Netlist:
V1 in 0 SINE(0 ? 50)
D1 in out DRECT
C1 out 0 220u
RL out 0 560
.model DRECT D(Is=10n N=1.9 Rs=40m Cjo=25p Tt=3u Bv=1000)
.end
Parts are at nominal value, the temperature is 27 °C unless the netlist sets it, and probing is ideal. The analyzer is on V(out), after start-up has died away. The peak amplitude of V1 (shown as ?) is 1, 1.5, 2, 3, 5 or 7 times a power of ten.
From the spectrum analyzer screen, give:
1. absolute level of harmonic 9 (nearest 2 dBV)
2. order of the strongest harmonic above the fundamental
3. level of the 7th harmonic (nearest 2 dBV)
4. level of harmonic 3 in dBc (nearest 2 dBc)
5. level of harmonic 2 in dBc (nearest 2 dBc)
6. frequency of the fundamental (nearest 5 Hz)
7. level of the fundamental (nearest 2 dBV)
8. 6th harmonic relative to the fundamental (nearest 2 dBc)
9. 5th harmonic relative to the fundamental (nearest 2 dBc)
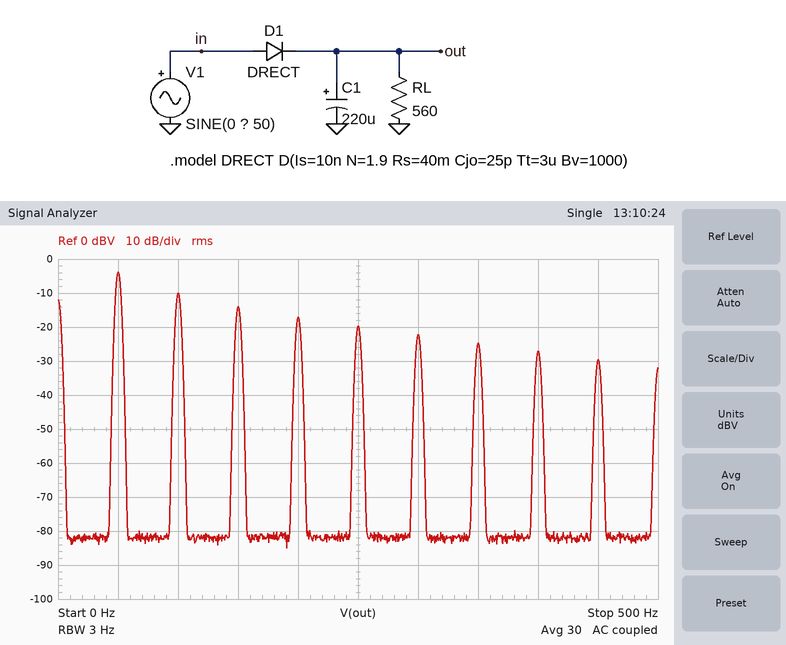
-30 dBV
2
-24 dBV
-10 dBc
-6 dBc
50 Hz
-4 dBV
-18 dBc
-16 dBc
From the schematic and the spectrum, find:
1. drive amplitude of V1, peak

20 V
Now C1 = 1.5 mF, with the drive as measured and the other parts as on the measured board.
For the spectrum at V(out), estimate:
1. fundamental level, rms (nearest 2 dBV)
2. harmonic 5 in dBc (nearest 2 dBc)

-20 dBV
-14 dBc
